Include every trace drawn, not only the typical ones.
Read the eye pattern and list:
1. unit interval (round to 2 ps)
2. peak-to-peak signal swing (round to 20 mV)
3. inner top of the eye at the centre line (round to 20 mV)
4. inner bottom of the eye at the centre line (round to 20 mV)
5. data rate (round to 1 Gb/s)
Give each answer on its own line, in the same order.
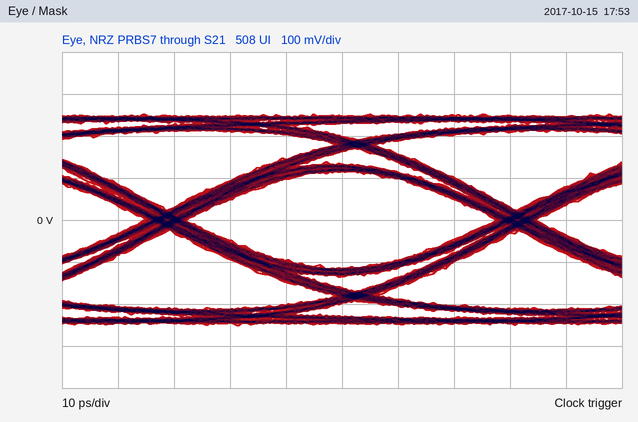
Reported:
62 ps
500 mV
120 mV
-120 mV
16 Gb/s
